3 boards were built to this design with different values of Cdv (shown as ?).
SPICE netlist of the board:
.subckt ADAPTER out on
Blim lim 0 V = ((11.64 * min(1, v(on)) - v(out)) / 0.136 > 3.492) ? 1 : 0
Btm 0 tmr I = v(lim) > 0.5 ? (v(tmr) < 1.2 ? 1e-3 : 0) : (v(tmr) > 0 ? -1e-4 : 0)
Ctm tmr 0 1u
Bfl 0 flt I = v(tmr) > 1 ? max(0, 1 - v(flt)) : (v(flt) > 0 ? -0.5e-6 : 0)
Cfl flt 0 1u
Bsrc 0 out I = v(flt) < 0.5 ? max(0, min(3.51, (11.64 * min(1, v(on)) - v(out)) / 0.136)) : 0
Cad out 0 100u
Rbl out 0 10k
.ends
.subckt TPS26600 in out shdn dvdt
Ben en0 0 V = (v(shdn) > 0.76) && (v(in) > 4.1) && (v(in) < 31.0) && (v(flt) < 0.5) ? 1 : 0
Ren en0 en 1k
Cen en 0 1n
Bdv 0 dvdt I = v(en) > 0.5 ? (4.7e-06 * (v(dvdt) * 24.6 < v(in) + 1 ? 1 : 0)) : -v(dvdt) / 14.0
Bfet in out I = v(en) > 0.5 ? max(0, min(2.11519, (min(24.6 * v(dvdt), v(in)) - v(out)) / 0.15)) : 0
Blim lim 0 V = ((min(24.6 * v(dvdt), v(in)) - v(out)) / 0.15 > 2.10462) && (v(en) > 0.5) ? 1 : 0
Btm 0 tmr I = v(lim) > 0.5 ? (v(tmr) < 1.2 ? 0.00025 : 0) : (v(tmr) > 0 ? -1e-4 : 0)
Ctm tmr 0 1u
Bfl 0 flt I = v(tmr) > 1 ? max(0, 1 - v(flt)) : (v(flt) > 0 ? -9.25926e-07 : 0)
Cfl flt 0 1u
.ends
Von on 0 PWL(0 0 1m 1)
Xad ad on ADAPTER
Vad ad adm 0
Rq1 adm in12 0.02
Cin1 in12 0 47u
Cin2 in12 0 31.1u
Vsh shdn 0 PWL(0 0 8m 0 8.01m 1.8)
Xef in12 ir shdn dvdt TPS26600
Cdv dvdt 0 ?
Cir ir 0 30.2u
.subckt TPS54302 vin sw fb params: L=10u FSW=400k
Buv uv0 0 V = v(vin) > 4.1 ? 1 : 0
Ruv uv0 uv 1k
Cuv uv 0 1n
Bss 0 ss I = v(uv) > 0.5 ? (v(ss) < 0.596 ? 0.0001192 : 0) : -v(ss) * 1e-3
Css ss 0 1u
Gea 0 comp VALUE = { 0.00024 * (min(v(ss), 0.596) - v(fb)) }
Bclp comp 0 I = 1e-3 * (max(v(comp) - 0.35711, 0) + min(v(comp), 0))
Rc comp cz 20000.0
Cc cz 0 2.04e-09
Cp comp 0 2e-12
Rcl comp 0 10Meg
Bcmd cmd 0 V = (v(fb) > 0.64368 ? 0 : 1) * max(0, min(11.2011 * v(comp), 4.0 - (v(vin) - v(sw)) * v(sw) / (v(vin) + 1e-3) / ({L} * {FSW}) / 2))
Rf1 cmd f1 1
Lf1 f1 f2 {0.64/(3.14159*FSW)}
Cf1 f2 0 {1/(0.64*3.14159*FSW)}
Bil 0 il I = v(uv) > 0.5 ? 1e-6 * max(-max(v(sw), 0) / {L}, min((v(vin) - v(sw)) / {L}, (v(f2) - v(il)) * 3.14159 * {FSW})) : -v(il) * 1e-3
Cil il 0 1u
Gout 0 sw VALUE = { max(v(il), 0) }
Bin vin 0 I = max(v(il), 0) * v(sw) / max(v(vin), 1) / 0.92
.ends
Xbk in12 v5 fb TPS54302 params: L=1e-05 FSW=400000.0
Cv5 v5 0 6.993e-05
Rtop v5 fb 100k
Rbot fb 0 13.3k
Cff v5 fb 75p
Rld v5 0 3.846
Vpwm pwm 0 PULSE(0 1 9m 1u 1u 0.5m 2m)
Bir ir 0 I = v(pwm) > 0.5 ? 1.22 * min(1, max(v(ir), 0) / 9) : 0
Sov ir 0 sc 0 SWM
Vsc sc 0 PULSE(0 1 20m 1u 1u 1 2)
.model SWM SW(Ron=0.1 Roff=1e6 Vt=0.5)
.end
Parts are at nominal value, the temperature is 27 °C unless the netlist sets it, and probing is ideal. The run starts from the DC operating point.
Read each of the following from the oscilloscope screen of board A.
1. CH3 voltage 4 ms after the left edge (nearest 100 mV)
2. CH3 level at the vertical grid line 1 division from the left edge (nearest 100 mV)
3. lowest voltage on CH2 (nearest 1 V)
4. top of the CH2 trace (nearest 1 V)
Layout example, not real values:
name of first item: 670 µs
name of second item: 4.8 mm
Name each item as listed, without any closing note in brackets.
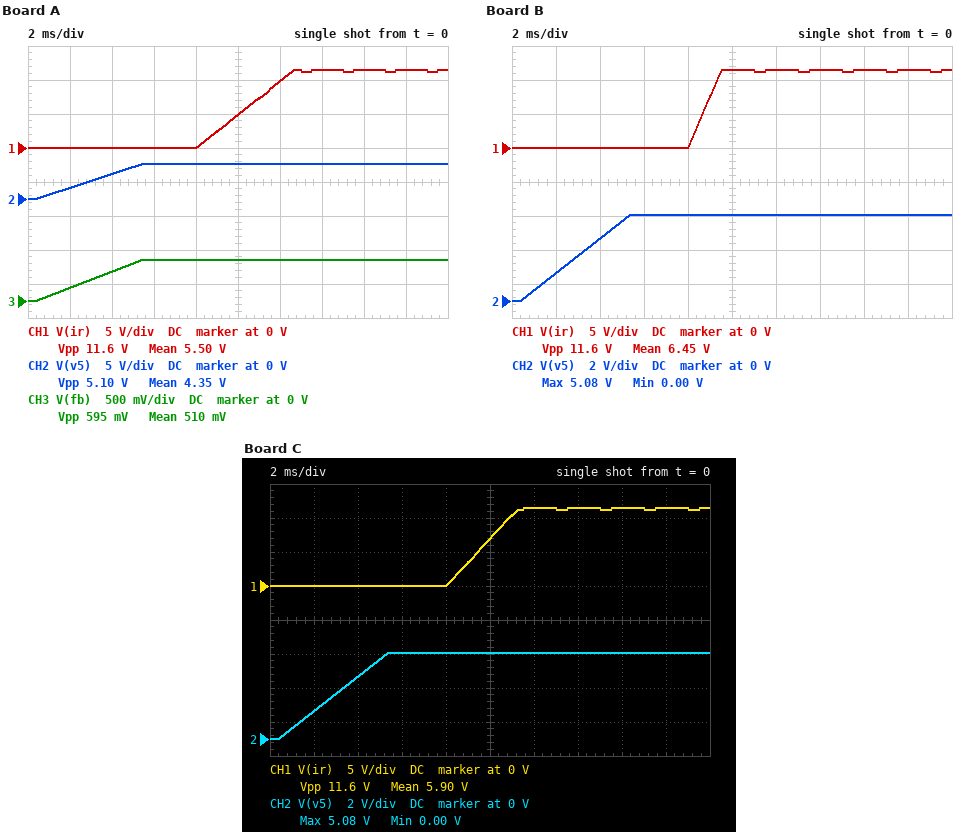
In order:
CH3 voltage 4 ms after the left edge: 400 mV
CH3 level at the vertical grid line 1 division from the left edge: 200 mV
lowest voltage on CH2: 0 V
top of the CH2 trace: 5 V
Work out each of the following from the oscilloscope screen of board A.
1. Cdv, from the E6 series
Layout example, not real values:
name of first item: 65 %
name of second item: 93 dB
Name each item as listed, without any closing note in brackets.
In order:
Cdv, from the E6 series: 47 nF
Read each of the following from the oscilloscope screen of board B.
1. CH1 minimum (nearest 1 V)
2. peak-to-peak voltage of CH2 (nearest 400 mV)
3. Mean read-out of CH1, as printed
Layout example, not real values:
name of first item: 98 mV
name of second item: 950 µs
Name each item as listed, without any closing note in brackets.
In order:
CH1 minimum: 0 V
peak-to-peak voltage of CH2: 5.2 V
Mean read-out of CH1, as printed: 6.45 V
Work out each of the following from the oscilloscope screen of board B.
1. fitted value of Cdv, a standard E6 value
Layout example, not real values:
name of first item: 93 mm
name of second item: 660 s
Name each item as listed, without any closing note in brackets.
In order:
fitted value of Cdv, a standard E6 value: 15 nF
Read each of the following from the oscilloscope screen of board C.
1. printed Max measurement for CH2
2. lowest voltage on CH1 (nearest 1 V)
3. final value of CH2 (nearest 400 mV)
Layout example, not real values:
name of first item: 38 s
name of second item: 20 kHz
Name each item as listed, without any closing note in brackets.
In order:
printed Max measurement for CH2: 5.08 V
lowest voltage on CH1: 0 V
final value of CH2: 5.2 V
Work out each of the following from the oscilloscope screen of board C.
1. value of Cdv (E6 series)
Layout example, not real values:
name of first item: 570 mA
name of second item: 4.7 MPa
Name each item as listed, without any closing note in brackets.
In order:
value of Cdv: 33 nF
